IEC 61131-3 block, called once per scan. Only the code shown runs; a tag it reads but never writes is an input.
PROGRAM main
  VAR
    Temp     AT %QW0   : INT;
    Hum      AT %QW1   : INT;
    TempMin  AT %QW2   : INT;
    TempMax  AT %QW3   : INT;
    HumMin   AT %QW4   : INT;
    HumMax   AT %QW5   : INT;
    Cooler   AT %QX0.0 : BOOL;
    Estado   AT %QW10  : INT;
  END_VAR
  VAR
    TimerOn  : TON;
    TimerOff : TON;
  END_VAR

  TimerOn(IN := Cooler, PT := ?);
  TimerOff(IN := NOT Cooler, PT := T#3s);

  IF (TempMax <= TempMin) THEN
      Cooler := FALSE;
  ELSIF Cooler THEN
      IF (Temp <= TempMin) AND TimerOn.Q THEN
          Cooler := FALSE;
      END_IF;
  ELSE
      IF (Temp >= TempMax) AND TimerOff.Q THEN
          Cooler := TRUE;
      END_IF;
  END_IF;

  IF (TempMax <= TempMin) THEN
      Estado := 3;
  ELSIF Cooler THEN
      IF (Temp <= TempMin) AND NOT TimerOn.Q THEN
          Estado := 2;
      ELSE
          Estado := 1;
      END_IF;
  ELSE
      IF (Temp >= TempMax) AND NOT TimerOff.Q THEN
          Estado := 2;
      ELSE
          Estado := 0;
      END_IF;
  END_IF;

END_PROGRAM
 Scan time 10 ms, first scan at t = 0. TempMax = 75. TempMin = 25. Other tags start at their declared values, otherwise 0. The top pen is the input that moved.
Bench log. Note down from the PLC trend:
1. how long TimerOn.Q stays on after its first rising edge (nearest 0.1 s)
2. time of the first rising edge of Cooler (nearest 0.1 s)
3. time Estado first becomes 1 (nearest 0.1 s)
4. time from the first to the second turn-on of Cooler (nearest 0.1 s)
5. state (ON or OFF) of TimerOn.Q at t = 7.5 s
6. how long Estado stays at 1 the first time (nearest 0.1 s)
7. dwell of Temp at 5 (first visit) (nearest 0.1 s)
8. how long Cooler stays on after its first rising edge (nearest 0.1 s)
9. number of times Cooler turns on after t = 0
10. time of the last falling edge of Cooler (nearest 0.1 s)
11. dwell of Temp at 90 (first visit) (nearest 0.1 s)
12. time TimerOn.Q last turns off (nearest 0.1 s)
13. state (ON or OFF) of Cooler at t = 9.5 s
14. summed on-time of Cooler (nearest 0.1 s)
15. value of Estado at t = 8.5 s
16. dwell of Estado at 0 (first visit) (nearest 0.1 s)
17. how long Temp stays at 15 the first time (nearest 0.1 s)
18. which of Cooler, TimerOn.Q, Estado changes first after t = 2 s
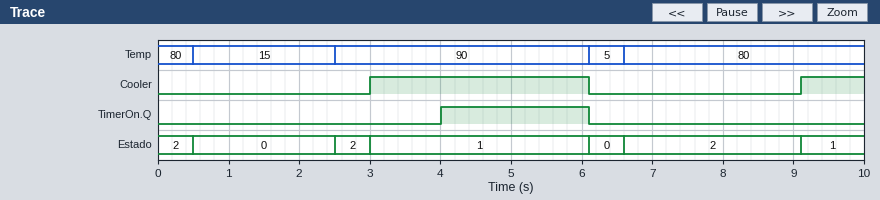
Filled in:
2.1 s
3.0 s
3.0 s
6.1 s
OFF
3.1 s
0.5 s
3.1 s
2
6.1 s
3.6 s
6.1 s
ON
4.0 s
2
2.0 s
2.0 s
Estado
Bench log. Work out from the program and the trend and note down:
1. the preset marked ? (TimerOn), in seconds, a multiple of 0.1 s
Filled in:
1.0 s
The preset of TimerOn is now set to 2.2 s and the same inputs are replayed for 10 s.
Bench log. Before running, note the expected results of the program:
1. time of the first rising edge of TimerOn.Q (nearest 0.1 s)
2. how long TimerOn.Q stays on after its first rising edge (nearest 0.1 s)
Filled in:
5.2 s
0.9 s
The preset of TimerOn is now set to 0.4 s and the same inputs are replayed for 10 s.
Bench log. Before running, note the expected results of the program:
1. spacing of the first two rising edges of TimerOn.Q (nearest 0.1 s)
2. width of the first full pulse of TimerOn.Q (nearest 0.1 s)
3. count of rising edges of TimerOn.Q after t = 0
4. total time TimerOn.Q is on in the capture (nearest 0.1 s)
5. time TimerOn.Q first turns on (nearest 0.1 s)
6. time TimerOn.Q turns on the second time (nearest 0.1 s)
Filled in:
6.1 s
2.7 s
2
3.2 s
3.4 s
9.5 s
